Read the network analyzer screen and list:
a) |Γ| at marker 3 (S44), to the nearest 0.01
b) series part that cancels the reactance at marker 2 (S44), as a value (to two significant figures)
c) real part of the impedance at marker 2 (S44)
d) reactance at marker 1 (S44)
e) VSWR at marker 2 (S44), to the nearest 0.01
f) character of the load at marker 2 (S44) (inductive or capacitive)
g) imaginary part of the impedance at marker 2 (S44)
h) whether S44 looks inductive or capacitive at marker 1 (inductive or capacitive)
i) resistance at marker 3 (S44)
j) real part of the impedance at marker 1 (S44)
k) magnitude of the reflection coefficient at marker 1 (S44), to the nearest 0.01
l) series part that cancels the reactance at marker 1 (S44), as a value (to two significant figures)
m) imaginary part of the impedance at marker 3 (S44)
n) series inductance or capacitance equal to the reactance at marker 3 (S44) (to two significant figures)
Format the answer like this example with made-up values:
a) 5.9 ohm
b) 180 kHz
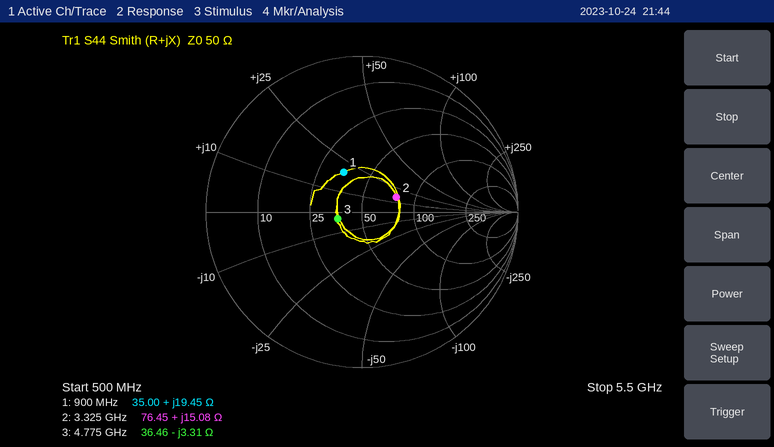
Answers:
a) 0.16
b) 3.2 pF
c) 76.45 Ω
d) +19.45 Ω
e) 1.63
f) inductive
g) +15.08 Ω
h) inductive
i) 36.46 Ω
j) 35.00 Ω
k) 0.28
l) 9.1 pF
m) -3.31 Ω
n) 10 pF
